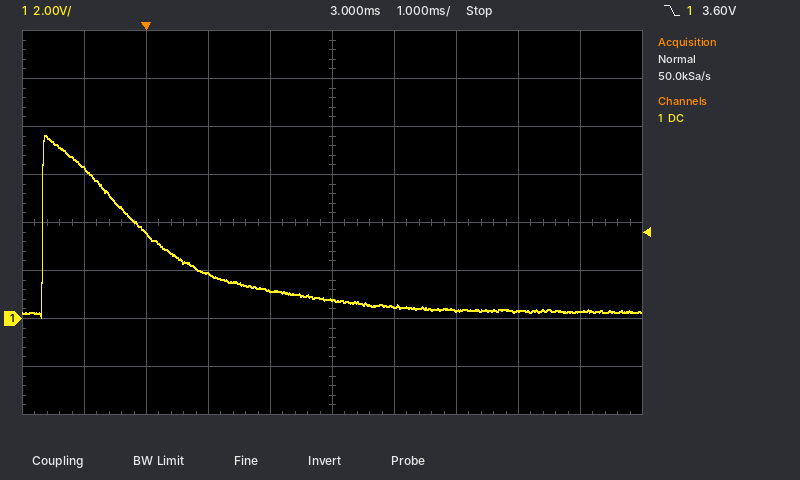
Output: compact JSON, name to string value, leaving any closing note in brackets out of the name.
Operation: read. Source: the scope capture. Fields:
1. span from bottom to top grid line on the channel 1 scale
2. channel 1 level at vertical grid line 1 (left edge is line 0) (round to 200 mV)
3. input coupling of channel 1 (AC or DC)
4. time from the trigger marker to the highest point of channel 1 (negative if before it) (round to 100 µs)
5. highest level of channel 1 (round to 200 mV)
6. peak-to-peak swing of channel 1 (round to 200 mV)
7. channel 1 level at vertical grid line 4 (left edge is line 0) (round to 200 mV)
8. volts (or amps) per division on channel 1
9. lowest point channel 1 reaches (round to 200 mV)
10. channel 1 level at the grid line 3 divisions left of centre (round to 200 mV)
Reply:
{"span from bottom to top grid line on the channel 1 scale": "16 V", "channel 1 level at vertical grid line 1 (left edge is line 0)": "6.2 V", "input coupling of channel 1": "DC", "time from the trigger marker to the highest point of channel 1 (negative if before it)": "-1.6 ms", "highest level of channel 1": "7.6 V", "peak-to-peak swing of channel 1": "7.6 V", "channel 1 level at vertical grid line 4 (left edge is line 0)": "1.2 V", "volts (or amps) per division on channel 1": "2 V", "lowest point channel 1 reaches": "0.0 V", "channel 1 level at the grid line 3 divisions left of centre": "3.6 V"}
